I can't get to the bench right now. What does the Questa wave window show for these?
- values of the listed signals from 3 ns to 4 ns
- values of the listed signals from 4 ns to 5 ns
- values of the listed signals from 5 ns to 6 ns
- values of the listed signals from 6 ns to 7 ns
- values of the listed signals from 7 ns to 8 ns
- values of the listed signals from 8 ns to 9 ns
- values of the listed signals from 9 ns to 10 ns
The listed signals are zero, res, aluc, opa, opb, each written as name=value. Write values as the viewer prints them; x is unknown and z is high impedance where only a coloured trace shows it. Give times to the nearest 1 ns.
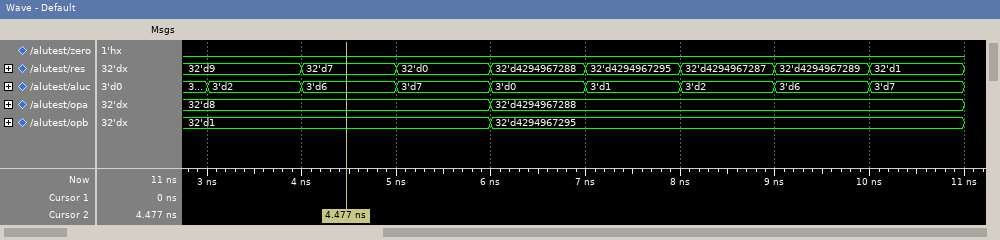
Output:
zero=0, res=32'd9, aluc=3'd2, opa=32'd8, opb=32'd1
zero=0, res=32'd7, aluc=3'd6, opa=32'd8, opb=32'd1
zero=0, res=32'd0, aluc=3'd7, opa=32'd8, opb=32'd1
zero=0, res=32'd4294967288, aluc=3'd0, opa=32'd4294967288, opb=32'd4294967295
zero=0, res=32'd4294967295, aluc=3'd1, opa=32'd4294967288, opb=32'd4294967295
zero=0, res=32'd4294967287, aluc=3'd2, opa=32'd4294967288, opb=32'd4294967295
zero=0, res=32'd4294967289, aluc=3'd6, opa=32'd4294967288, opb=32'd4294967295
